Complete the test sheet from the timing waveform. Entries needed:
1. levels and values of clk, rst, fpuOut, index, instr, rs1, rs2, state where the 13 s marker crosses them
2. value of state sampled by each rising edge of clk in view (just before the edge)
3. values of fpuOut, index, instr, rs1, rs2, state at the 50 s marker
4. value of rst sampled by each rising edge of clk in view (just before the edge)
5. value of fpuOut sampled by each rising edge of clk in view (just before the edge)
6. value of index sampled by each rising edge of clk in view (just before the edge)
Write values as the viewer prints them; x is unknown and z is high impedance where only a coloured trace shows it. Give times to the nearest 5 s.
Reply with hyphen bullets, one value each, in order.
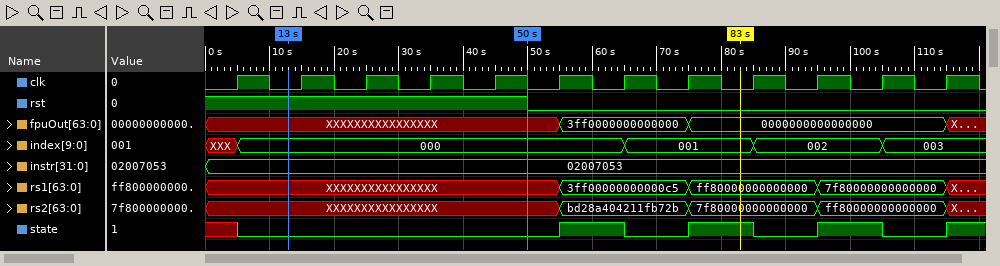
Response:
- clk=0, rst=1, fpuOut=XXXXXXXXXXXXXXXX, index=000, instr=02007053, rs1=XXXXXXXXXXXXXXXX, rs2=XXXXXXXXXXXXXXXX, state=0
- x 0 0 0 0 0 1 0 1 0 1 0
- fpuOut=XXXXXXXXXXXXXXXX, index=000, instr=02007053, rs1=XXXXXXXXXXXXXXXX, rs2=XXXXXXXXXXXXXXXX, state=0
- 1 1 1 1 1 0 0 0 0 0 0 0
- XXXXXXXXXXXXXXXX, XXXXXXXXXXXXXXXX, XXXXXXXXXXXXXXXX, XXXXXXXXXXXXXXXX, XXXXXXXXXXXXXXXX, XXXXXXXXXXXXXXXX, 3ff0000000000000, 3ff0000000000000, 0000000000000000, 0000000000000000, 0000000000000000, 0000000000000000
- XXX, 000, 000, 000, 000, 000, 000, 001, 001, 002, 002, 003
